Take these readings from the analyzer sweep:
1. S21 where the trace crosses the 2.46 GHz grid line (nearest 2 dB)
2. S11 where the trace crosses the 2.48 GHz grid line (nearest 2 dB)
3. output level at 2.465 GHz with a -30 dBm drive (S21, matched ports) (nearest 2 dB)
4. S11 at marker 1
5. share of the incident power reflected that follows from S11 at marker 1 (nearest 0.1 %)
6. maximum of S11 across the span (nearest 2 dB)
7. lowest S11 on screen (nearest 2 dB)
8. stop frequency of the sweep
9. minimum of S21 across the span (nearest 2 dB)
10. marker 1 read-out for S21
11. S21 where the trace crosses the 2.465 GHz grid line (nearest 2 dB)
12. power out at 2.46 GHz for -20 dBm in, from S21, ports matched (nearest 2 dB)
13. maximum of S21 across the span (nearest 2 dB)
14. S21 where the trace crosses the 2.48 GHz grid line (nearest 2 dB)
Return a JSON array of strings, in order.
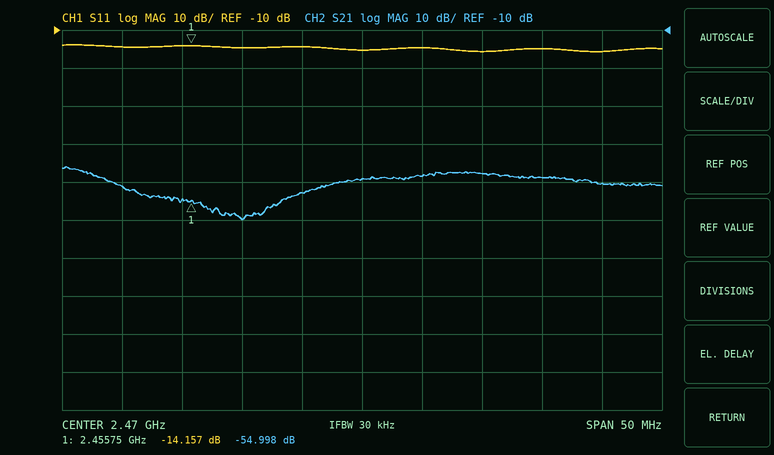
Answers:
["-60 dB", "-16 dB", "-82 dBm", "-14.157 dB", "3.8 %", "-14 dB", "-16 dB", "2.495 GHz", "-60 dB", "-54.998 dB", "-52 dB", "-80 dBm", "-46 dB", "-48 dB"]
